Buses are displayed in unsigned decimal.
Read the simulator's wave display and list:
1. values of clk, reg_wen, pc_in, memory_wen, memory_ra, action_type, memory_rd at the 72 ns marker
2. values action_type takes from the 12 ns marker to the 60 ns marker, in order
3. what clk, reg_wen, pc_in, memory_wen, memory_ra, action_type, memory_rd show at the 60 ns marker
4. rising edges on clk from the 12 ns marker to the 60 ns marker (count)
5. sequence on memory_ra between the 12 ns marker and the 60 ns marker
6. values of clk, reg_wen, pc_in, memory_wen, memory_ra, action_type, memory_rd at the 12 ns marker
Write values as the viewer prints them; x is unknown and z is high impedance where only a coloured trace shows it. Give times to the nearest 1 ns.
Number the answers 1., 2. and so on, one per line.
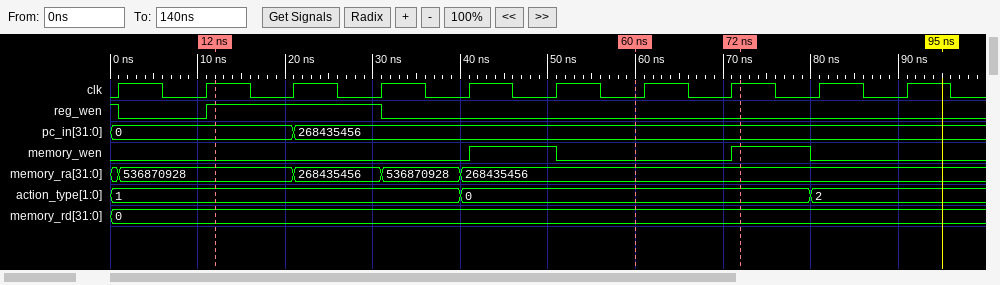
1. clk=1, reg_wen=0, pc_in=268435456, memory_wen=1, memory_ra=268435456, action_type=0, memory_rd=0
2. 1, 0
3. clk=0, reg_wen=0, pc_in=268435456, memory_wen=0, memory_ra=268435456, action_type=0, memory_rd=0
4. 4
5. 536870928, 268435456, 536870928, 268435456
6. clk=1, reg_wen=1, pc_in=0, memory_wen=0, memory_ra=536870928, action_type=1, memory_rd=0
